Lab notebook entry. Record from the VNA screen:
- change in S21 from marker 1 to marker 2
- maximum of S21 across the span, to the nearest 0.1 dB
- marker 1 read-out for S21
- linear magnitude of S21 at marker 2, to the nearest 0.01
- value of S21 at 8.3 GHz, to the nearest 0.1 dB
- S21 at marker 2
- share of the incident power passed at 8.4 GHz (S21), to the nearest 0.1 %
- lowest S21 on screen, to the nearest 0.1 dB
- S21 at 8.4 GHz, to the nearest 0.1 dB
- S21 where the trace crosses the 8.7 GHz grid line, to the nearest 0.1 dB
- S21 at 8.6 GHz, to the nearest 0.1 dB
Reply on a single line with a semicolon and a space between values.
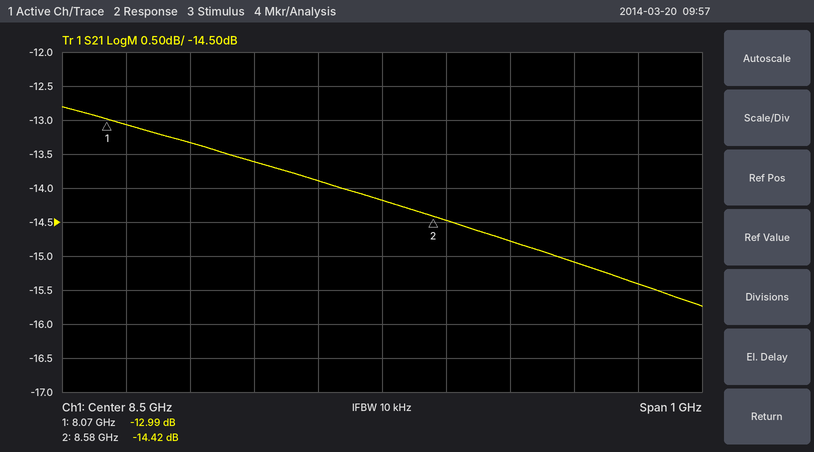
-1.43 dB; -12.8 dB; -12.99 dB; 0.19; -13.6 dB; -14.42 dB; 4.1 %; -15.7 dB; -13.9 dB; -14.8 dB; -14.5 dB
